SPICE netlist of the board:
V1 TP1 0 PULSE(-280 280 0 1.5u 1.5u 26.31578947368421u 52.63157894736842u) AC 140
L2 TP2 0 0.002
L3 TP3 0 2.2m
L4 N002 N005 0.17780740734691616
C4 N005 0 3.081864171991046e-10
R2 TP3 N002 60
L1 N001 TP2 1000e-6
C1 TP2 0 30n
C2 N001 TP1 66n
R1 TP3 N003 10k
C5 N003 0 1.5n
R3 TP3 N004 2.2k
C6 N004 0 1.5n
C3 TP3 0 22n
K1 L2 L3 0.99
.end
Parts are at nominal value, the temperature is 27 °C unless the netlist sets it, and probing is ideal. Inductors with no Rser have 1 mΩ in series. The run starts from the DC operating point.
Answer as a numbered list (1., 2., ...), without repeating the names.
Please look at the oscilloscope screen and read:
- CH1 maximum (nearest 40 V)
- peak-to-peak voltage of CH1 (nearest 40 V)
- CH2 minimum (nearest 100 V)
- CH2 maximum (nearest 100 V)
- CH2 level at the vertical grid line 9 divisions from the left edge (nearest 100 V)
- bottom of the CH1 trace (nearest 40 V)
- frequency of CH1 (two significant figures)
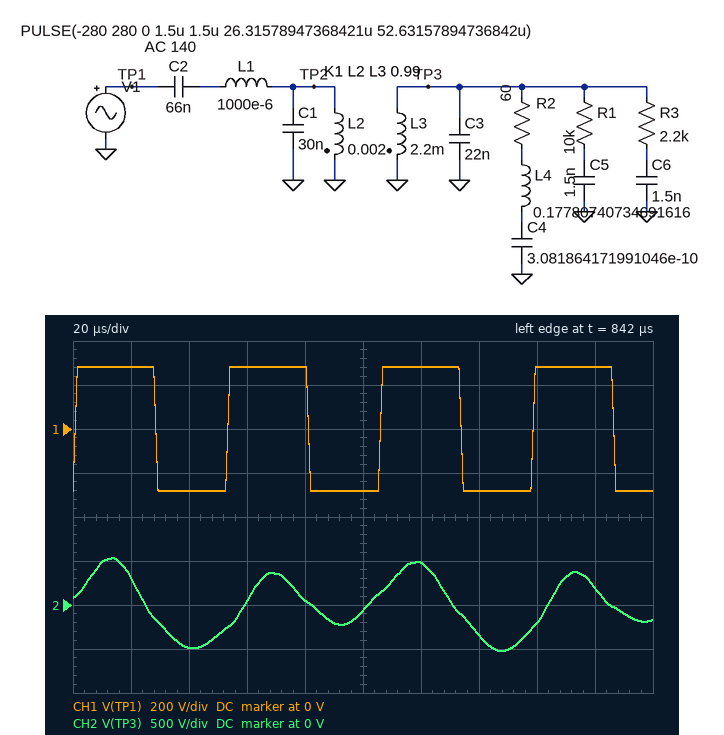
1. 280 V
2. 560 V
3. -500 V
4. 500 V
5. 200 V
6. -280 V
7. 19 kHz
